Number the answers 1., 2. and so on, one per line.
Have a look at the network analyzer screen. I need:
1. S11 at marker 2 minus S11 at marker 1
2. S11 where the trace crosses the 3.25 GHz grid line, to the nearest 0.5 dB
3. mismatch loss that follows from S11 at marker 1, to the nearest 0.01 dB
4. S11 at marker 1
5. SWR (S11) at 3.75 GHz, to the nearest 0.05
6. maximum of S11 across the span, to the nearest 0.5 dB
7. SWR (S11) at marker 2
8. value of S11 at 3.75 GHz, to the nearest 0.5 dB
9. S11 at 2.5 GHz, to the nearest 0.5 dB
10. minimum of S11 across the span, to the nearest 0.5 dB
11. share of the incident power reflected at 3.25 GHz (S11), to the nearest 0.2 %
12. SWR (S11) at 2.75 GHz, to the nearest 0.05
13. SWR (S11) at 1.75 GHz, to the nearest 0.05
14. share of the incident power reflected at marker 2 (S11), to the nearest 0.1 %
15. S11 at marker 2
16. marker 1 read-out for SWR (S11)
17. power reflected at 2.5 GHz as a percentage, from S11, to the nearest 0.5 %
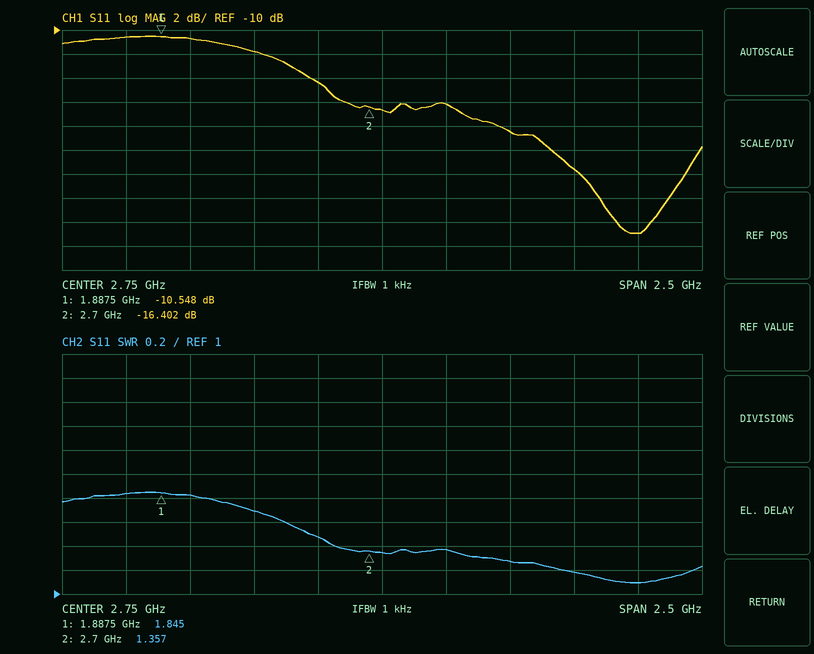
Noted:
1. -5.854 dB
2. -18.5 dB
3. 0.40 dB
4. -10.548 dB
5. 1.10
6. -10.5 dB
7. 1.357
8. -27.0 dB
9. -14.5 dB
10. -27.0 dB
11. 1.4 %
12. 1.35
13. 1.85
14. 2.3 %
15. -16.402 dB
16. 1.845
17. 3.5 %
